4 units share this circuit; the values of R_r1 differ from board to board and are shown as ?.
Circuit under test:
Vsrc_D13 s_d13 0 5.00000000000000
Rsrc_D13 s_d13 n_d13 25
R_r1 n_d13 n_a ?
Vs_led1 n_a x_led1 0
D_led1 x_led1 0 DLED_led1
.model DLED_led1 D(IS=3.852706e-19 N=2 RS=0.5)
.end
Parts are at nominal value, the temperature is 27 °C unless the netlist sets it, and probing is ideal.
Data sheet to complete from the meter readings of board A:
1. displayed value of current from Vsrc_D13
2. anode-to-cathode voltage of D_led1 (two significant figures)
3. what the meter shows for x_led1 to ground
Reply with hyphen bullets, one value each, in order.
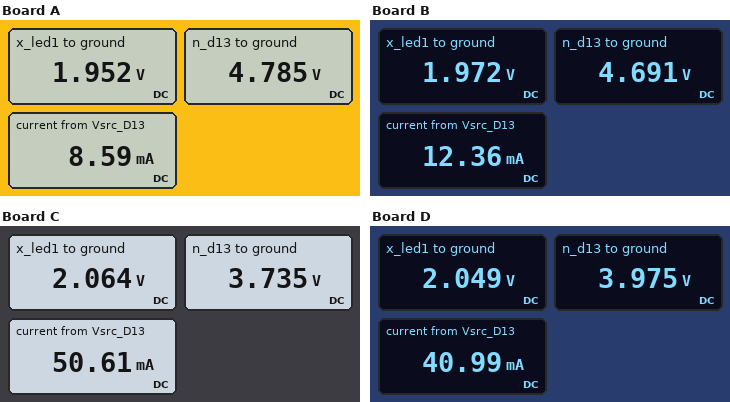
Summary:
- 8.59 mA
- 2.0 V
- 1.952 V
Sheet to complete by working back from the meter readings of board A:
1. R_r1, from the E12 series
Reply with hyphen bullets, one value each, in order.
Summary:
- 330 Ω
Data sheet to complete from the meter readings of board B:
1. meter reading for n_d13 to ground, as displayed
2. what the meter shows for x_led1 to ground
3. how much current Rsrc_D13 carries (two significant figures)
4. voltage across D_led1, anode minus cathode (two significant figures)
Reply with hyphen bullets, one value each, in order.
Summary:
- 4.691 V
- 1.972 V
- 12 mA
- 2.0 V
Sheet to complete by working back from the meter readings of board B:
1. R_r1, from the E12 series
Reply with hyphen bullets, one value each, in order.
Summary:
- 220 Ω
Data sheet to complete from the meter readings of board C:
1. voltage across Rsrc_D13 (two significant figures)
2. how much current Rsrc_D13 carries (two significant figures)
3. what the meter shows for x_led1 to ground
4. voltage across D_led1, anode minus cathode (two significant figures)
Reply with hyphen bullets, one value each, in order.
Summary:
- 1.3 V
- 51 mA
- 2.064 V
- 2.1 V
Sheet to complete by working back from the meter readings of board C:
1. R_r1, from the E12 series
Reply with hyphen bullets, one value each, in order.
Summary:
- 33 Ω
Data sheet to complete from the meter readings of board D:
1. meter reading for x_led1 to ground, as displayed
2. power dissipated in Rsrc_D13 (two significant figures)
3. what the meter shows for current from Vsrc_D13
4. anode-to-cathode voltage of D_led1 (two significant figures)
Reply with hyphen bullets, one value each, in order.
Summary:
- 2.049 V
- 42 mW
- 40.99 mA
- 2.0 V
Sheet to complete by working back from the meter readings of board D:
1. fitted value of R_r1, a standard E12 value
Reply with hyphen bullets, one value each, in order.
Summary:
- 47 Ω
